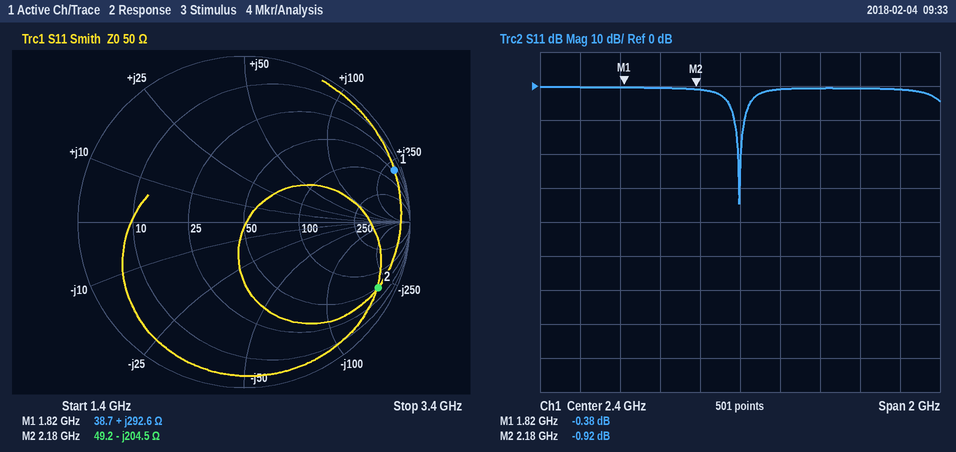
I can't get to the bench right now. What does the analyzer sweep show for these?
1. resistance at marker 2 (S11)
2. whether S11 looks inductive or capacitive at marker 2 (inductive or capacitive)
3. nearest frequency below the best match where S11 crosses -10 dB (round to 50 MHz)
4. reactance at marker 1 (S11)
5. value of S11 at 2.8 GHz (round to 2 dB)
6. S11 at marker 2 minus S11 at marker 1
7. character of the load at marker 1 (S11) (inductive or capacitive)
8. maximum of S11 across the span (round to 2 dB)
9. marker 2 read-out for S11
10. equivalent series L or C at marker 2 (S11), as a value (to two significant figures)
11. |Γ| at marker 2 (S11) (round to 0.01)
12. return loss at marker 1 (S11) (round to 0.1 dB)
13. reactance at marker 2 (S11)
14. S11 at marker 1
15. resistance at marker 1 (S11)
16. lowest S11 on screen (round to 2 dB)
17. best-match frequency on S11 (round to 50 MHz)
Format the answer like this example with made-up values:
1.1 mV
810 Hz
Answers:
49.2 Ω
capacitive
2.35 GHz
+292.6 Ω
0 dB
-0.54 dB
inductive
0 dB
-0.92 dB
360 fF
0.90
0.4 dB
-204.5 Ω
-0.38 dB
38.7 Ω
-34 dB
2.40 GHz
